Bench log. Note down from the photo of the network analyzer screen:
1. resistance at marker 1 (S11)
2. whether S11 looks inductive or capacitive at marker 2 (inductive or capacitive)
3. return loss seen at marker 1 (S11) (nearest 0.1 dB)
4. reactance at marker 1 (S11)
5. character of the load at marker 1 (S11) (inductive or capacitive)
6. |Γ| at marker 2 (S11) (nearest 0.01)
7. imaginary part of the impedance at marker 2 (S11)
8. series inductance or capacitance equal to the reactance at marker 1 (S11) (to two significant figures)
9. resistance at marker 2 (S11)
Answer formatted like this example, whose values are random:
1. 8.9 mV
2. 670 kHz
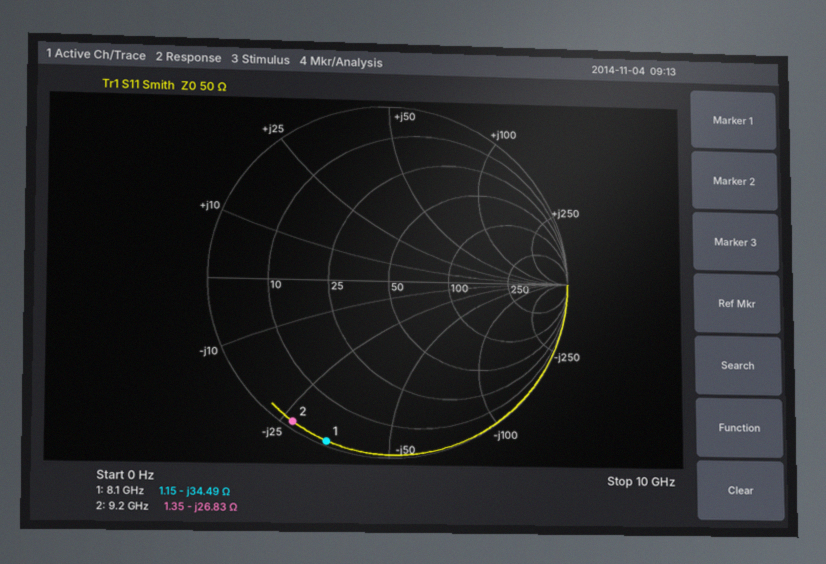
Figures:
1. 1.15 Ω
2. capacitive
3. 0.3 dB
4. -34.49 Ω
5. capacitive
6. 0.96
7. -26.83 Ω
8. 570 fF
9. 1.35 Ω
